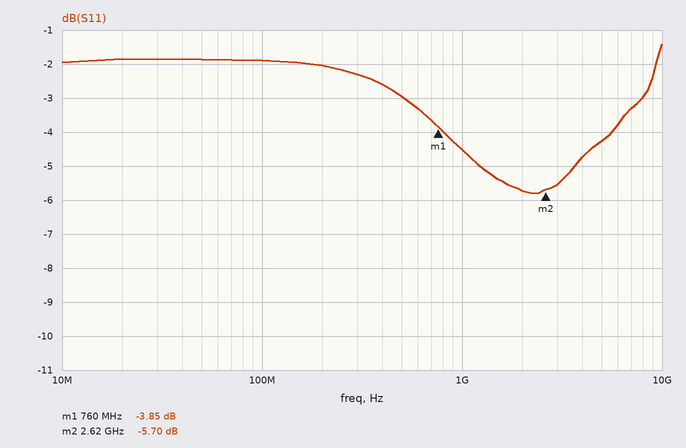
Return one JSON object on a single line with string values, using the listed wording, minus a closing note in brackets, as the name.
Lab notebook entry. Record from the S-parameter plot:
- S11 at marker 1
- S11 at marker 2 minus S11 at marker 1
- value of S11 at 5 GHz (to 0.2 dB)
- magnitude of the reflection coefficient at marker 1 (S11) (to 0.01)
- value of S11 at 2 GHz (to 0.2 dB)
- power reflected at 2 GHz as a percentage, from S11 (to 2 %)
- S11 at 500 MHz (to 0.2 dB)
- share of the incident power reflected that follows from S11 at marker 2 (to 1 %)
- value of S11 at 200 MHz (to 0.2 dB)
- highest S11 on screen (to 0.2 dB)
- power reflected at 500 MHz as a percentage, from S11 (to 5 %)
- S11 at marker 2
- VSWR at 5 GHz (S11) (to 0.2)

{"S11 at marker 1": "-3.85 dB", "S11 at marker 2 minus S11 at marker 1": "-1.85 dB", "value of S11 at 5 GHz": "-4.2 dB", "magnitude of the reflection coefficient at marker 1 (S11)": "0.64", "value of S11 at 2 GHz": "-5.8 dB", "power reflected at 2 GHz as a percentage, from S11": "26 %", "S11 at 500 MHz": "-3.0 dB", "share of the incident power reflected that follows from S11 at marker 2": "27 %", "value of S11 at 200 MHz": "-2.0 dB", "highest S11 on screen": "-1.4 dB", "power reflected at 500 MHz as a percentage, from S11": "50 %", "S11 at marker 2": "-5.70 dB", "VSWR at 5 GHz (S11)": "4.2"}
